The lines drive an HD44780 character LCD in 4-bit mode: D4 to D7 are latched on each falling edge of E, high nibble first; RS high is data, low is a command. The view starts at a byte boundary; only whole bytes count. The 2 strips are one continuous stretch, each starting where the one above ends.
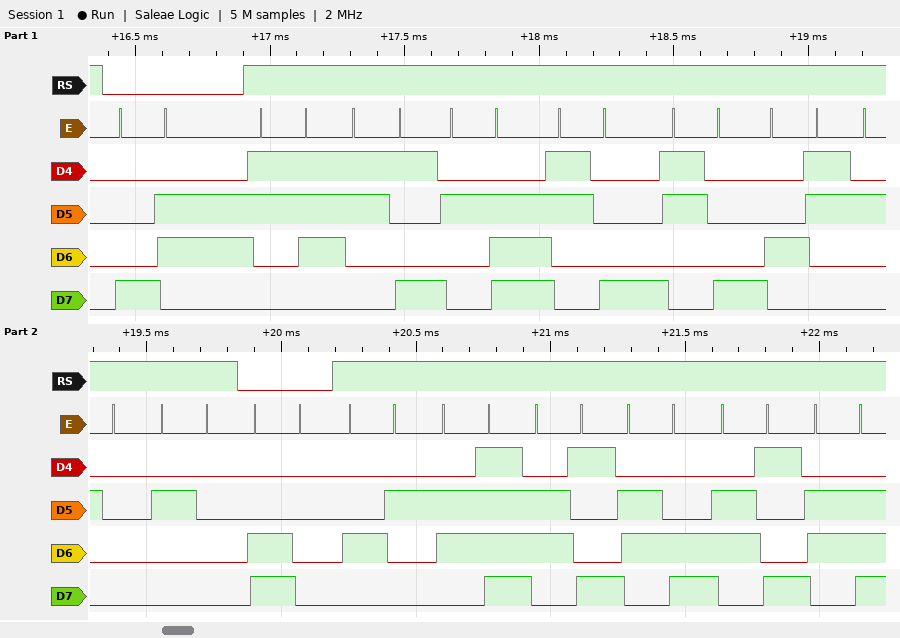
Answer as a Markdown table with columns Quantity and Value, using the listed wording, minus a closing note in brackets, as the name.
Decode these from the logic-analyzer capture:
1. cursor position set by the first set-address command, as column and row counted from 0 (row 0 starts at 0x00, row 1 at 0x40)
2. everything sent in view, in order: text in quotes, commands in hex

| Quantity | Value |
|---|---|
| cursor position set by the first set-address command, as column and row counted from 0 | column 6, row 0 |
| everything sent in view, in order: text in quotes, commands in hex | 0x86 "79.88C  " 0xC0 "Boilin" |
